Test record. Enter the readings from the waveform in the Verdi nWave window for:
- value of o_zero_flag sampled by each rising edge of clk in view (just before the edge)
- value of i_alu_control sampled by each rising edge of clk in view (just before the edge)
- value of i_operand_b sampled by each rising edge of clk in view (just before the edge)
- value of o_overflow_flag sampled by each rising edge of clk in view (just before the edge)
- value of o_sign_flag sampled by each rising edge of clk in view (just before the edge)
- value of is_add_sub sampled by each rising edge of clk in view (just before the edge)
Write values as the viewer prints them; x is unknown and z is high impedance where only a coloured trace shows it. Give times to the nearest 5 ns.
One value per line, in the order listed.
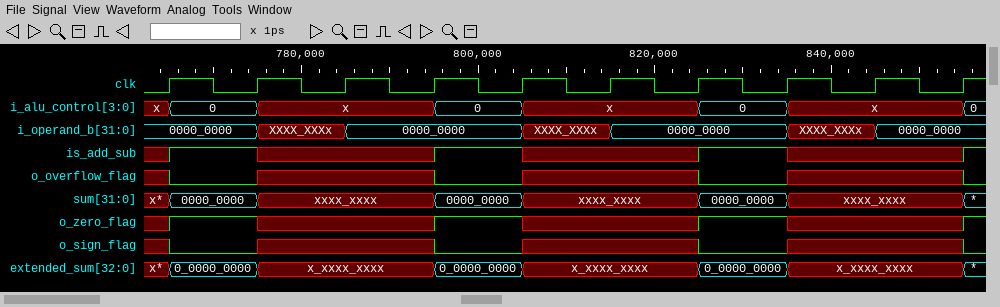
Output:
x 1 x x 1 x x 1 x x
x, 0, x, x, 0, x, x, 0, x, x
0000_0000, 0000_0000, XXXX_XXXx, 0000_0000, 0000_0000, XXXX_XXXx, 0000_0000, 0000_0000, XXXX_XXXx, 0000_0000
x 0 x x 0 x x 0 x x
x 0 x x 0 x x 0 x x
x 1 x x 1 x x 1 x x
